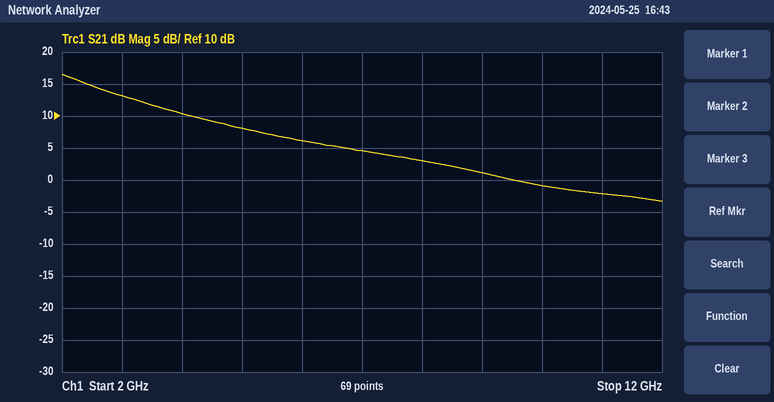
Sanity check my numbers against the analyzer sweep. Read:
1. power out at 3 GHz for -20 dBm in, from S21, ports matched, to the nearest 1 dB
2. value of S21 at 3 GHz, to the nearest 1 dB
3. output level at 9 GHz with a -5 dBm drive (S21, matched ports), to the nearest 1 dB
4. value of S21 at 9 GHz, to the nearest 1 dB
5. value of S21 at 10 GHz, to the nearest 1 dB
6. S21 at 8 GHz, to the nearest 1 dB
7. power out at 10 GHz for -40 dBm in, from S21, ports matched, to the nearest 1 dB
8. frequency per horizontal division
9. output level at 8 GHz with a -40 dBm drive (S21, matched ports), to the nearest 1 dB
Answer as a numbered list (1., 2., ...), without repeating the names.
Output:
1. -7 dBm
2. 13 dB
3. -4 dBm
4. 1 dB
5. -1 dB
6. 3 dB
7. -41 dBm
8. 1 GHz
9. -37 dBm
